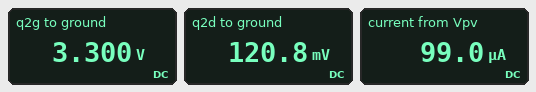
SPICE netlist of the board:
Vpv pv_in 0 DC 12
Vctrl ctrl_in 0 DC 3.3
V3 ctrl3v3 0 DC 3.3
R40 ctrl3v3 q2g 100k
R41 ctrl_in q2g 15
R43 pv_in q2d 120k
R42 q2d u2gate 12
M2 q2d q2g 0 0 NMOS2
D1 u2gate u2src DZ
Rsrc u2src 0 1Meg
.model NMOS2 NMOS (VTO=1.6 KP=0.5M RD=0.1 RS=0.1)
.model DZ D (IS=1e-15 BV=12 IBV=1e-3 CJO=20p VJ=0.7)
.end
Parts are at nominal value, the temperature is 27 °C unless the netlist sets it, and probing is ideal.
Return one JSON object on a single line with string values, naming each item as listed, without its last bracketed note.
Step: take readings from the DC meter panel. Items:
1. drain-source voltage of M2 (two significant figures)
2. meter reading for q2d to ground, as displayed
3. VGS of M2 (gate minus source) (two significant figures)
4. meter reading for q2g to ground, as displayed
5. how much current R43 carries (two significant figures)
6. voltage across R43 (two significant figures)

{"drain-source voltage of M2": "120 mV", "meter reading for q2d to ground, as displayed": "120.8 mV", "VGS of M2 (gate minus source)": "3.3 V", "meter reading for q2g to ground, as displayed": "3.300 V", "how much current R43 carries": "99 µA", "voltage across R43": "12 V"}
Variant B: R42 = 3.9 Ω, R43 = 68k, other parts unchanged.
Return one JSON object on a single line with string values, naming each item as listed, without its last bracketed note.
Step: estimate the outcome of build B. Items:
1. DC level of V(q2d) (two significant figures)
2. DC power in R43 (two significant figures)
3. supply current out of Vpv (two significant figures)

{"DC level of V(q2d)": "220 mV", "DC power in R43": "2.0 mW", "supply current out of Vpv": "170 µA"}
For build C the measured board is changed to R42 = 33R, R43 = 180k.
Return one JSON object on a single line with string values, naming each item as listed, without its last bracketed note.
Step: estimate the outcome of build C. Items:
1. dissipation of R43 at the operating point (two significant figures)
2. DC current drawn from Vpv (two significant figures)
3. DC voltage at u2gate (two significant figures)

{"dissipation of R43 at the operating point": "790 µW", "DC current drawn from Vpv": "66 µA", "DC voltage at u2gate": "80 mV"}
